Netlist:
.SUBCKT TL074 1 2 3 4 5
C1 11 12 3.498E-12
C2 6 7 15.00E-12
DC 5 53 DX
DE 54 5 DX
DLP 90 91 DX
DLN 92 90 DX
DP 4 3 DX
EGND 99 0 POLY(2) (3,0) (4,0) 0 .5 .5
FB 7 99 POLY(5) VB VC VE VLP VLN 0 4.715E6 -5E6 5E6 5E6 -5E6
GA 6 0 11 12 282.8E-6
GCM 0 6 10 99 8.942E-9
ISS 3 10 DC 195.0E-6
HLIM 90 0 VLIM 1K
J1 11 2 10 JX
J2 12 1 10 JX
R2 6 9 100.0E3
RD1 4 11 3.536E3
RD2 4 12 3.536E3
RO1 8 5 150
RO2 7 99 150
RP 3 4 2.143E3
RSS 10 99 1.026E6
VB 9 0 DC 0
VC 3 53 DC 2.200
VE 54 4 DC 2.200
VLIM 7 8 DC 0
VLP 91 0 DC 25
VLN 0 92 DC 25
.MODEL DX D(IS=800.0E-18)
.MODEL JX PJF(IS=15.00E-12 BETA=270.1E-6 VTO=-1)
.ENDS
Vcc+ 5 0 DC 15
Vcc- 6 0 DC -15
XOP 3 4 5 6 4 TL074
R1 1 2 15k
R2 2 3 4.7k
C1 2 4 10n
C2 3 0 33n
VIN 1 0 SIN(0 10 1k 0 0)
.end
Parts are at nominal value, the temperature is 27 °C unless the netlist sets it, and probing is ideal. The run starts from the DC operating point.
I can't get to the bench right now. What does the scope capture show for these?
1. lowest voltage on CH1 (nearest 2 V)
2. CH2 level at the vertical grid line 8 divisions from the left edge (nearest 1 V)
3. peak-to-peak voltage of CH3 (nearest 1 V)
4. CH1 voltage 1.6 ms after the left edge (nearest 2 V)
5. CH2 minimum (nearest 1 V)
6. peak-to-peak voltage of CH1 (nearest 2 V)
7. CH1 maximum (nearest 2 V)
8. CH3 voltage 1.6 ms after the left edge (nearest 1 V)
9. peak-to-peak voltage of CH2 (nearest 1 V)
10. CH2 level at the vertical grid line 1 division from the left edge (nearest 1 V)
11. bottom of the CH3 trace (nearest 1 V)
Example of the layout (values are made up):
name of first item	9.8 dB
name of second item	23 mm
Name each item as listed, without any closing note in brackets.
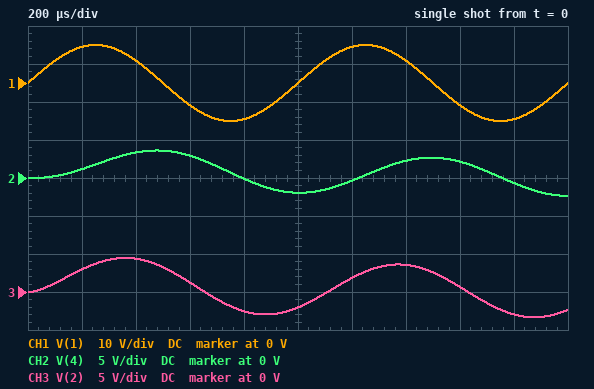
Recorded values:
lowest voltage on CH1	-10 V
CH2 level at the vertical grid line 8 divisions from the left edge	2 V
peak-to-peak voltage of CH3	8 V
CH1 voltage 1.6 ms after the left edge	-6 V
CH2 minimum	-2 V
peak-to-peak voltage of CH1	20 V
CH1 maximum	10 V
CH3 voltage 1.6 ms after the left edge	1 V
peak-to-peak voltage of CH2	6 V
CH2 level at the vertical grid line 1 division from the left edge	1 V
bottom of the CH3 trace	-3 V
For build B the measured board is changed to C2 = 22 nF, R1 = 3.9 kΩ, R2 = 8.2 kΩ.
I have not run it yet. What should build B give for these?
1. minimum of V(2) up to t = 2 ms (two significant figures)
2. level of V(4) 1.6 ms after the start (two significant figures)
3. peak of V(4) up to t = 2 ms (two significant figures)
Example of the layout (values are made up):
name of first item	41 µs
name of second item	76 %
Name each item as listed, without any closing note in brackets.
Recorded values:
minimum of V(2) up to t = 2 ms	-8.3 V
level of V(4) 1.6 ms after the start	2.8 V
peak of V(4) up to t = 2 ms	6.4 V
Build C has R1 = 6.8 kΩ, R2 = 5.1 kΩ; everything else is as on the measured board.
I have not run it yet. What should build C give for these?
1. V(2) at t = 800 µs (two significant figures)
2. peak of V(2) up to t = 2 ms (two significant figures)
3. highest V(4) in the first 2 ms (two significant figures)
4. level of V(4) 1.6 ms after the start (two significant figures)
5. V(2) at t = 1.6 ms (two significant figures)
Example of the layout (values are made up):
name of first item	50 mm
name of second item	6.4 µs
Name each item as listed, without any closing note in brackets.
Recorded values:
V(2) at t = 800 µs	-5.4 V
peak of V(2) up to t = 2 ms	6.6 V
highest V(4) in the first 2 ms	5.1 V
level of V(4) 1.6 ms after the start	2.7 V
V(2) at t = 1.6 ms	-490 mV
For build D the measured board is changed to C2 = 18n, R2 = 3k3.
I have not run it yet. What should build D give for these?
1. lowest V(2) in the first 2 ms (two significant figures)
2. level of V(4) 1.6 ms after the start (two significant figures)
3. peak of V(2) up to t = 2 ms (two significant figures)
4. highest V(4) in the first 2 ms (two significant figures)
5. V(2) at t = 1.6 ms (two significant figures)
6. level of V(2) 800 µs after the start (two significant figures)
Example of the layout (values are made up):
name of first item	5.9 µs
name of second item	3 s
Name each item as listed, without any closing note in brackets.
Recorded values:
lowest V(2) in the first 2 ms	-4.9 V
level of V(4) 1.6 ms after the start	2.8 V
peak of V(2) up to t = 2 ms	5.9 V
highest V(4) in the first 2 ms	5.7 V
V(2) at t = 1.6 ms	1.4 V
level of V(2) 800 µs after the start	-3.8 V
